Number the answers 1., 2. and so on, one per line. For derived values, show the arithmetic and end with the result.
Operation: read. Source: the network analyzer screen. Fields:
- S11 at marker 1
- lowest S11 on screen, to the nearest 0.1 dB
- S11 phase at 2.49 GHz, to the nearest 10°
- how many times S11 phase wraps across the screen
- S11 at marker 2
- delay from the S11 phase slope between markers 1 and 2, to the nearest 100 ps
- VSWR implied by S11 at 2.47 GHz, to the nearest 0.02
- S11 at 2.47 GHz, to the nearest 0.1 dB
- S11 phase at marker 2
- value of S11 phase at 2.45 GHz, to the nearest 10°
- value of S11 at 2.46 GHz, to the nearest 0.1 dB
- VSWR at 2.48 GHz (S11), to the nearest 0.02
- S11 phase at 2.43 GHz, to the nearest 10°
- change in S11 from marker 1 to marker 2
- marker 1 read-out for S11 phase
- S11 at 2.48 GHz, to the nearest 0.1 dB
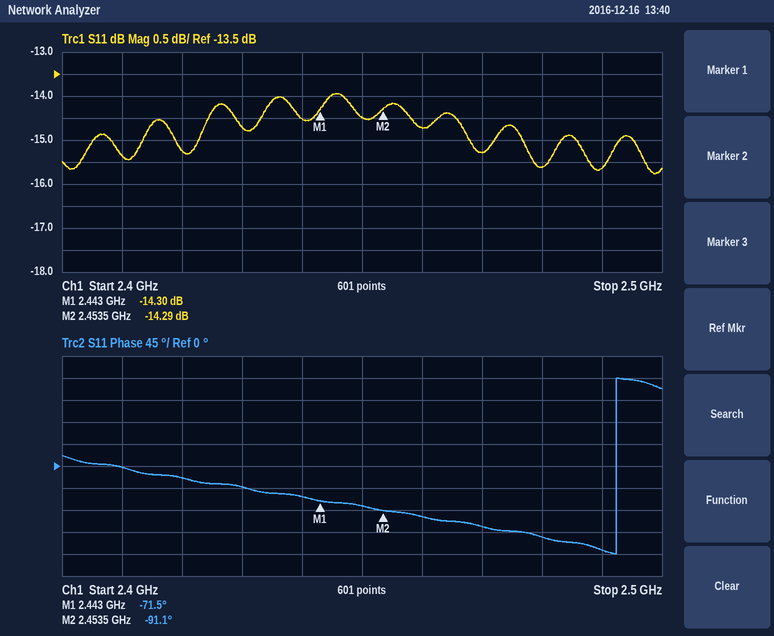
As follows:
1. -14.30 dB
2. -15.8 dB
3. -170°
4. 1
5. -14.29 dB
6. −(-91.1° − (-71.5°))/(360° × 10.5 MHz) ≈ 5.2 ns
7. |Γ| = 10^(-15.3/20) = 0.1718; VSWR = (1 + 0.1718)/(1 − 0.1718) ≈ 1.41, so 1.42 to the nearest 0.02
8. -15.3 dB
9. -91.1°
10. -80°
11. -14.7 dB
12. |Γ| = 10^(-15.6/20) = 0.1660; VSWR = (1 + 0.1660)/(1 − 0.1660) ≈ 1.40
13. -40°
14. -14.29 − (-14.3) = 0.01 dB
15. -71.5°
16. -15.6 dB
